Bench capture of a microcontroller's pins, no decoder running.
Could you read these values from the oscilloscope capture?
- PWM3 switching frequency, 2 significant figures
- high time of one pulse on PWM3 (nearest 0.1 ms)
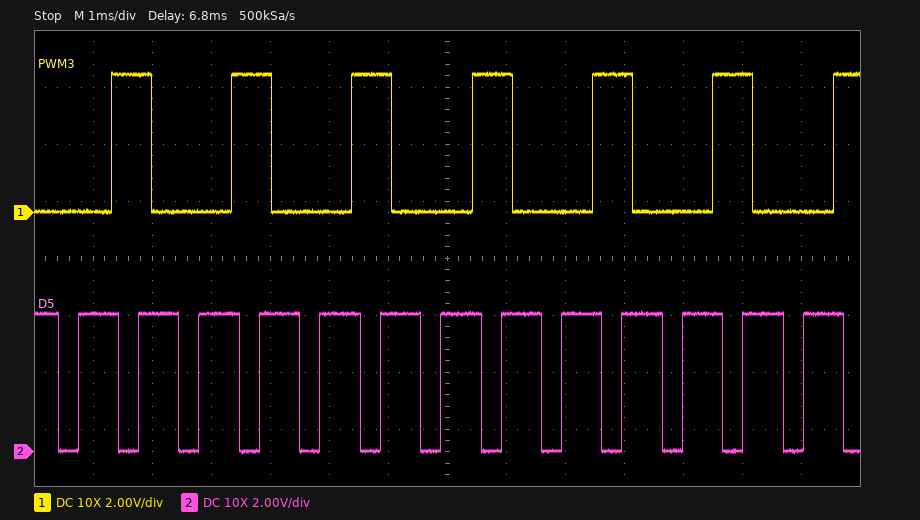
490 Hz
0.7 ms
